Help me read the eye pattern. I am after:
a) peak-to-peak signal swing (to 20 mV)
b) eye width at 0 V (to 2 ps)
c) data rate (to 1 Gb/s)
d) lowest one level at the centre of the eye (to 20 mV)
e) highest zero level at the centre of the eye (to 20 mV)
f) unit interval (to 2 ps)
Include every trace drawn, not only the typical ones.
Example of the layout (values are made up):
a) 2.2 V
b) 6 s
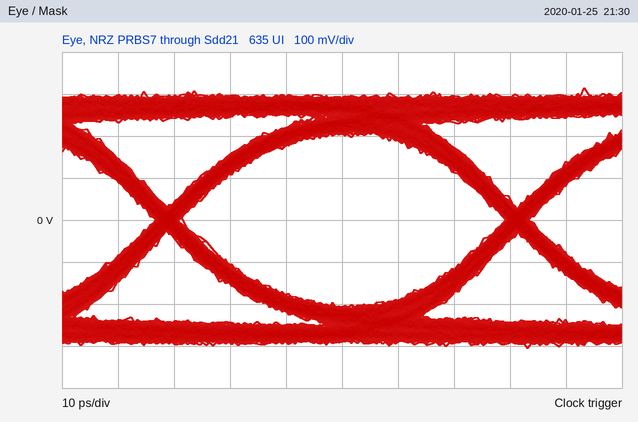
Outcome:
a) 620 mV
b) 58 ps
c) 16 Gb/s
d) 200 mV
e) -200 mV
f) 62 ps
